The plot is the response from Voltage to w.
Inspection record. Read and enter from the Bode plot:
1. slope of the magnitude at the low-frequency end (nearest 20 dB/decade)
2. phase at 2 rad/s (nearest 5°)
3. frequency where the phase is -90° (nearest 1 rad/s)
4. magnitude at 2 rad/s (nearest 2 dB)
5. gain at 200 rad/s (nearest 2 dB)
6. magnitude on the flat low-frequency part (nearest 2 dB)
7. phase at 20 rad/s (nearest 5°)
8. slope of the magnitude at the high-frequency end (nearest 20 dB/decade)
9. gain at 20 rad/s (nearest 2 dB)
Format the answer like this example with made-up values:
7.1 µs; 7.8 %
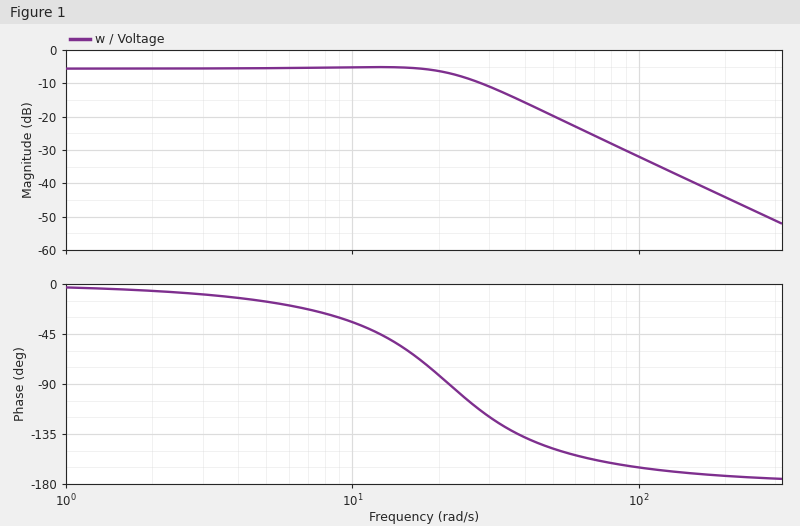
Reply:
0 dB/decade; -5°; 22 rad/s; -6 dB; -44 dB; -6 dB; -80°; -40 dB/decade; -6 dB
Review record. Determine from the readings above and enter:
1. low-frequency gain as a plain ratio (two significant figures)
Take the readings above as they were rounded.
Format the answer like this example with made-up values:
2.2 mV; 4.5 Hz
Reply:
0.50
